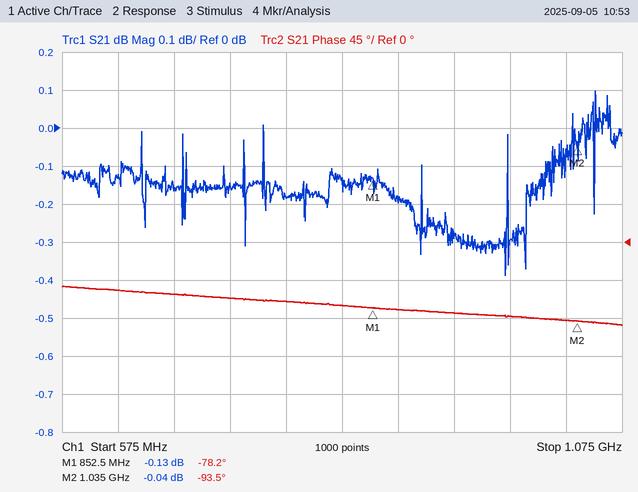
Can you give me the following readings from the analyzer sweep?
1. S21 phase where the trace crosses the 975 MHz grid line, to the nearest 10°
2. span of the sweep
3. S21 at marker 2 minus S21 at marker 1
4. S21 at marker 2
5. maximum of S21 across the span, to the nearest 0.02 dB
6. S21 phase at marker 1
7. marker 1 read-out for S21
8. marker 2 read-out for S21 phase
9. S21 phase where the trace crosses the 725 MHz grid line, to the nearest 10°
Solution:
-90°
500 MHz
0.09 dB
-0.04 dB
0.10 dB
-78.2°
-0.13 dB
-93.5°
-70°
